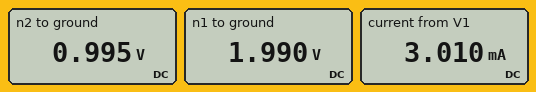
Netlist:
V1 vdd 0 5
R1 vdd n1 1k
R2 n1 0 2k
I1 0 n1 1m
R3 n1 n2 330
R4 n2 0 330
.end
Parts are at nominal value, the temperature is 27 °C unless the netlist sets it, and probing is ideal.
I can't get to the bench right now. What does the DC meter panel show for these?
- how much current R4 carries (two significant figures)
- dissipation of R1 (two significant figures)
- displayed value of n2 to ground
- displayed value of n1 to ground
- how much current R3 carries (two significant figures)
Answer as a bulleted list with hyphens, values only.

- 3.0 mA
- 9.1 mW
- 0.995 V
- 1.990 V
- 3.0 mA
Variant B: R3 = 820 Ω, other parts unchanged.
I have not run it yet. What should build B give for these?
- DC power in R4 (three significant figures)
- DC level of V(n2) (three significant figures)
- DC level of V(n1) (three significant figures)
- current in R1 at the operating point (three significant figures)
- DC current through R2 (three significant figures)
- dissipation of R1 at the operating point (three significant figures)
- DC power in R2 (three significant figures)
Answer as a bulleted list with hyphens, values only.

- 1.60 mW
- 727 mV
- 2.53 V
- 2.47 mA
- 1.27 mA
- 6.09 mW
- 3.21 mW
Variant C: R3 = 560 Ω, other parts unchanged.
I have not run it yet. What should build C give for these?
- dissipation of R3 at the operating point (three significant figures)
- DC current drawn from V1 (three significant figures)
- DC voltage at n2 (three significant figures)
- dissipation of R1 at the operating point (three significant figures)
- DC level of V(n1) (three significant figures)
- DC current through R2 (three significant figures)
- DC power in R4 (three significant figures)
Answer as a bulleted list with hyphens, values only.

- 3.70 mW
- 2.71 mA
- 848 mV
- 7.36 mW
- 2.29 V
- 1.14 mA
- 2.18 mW
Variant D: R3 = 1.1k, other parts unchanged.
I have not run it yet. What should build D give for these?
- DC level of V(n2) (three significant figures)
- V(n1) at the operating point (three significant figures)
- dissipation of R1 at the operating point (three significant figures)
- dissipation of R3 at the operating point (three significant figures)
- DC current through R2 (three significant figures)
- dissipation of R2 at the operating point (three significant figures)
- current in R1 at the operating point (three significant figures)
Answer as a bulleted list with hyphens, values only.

- 630 mV
- 2.73 V
- 5.16 mW
- 4.00 mW
- 1.36 mA
- 3.72 mW
- 2.27 mA
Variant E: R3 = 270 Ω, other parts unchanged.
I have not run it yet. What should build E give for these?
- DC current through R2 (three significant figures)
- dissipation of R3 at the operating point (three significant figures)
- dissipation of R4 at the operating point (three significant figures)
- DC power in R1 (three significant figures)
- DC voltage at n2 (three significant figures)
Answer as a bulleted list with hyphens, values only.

- 947 µA
- 2.69 mW
- 3.29 mW
- 9.64 mW
- 1.04 V
